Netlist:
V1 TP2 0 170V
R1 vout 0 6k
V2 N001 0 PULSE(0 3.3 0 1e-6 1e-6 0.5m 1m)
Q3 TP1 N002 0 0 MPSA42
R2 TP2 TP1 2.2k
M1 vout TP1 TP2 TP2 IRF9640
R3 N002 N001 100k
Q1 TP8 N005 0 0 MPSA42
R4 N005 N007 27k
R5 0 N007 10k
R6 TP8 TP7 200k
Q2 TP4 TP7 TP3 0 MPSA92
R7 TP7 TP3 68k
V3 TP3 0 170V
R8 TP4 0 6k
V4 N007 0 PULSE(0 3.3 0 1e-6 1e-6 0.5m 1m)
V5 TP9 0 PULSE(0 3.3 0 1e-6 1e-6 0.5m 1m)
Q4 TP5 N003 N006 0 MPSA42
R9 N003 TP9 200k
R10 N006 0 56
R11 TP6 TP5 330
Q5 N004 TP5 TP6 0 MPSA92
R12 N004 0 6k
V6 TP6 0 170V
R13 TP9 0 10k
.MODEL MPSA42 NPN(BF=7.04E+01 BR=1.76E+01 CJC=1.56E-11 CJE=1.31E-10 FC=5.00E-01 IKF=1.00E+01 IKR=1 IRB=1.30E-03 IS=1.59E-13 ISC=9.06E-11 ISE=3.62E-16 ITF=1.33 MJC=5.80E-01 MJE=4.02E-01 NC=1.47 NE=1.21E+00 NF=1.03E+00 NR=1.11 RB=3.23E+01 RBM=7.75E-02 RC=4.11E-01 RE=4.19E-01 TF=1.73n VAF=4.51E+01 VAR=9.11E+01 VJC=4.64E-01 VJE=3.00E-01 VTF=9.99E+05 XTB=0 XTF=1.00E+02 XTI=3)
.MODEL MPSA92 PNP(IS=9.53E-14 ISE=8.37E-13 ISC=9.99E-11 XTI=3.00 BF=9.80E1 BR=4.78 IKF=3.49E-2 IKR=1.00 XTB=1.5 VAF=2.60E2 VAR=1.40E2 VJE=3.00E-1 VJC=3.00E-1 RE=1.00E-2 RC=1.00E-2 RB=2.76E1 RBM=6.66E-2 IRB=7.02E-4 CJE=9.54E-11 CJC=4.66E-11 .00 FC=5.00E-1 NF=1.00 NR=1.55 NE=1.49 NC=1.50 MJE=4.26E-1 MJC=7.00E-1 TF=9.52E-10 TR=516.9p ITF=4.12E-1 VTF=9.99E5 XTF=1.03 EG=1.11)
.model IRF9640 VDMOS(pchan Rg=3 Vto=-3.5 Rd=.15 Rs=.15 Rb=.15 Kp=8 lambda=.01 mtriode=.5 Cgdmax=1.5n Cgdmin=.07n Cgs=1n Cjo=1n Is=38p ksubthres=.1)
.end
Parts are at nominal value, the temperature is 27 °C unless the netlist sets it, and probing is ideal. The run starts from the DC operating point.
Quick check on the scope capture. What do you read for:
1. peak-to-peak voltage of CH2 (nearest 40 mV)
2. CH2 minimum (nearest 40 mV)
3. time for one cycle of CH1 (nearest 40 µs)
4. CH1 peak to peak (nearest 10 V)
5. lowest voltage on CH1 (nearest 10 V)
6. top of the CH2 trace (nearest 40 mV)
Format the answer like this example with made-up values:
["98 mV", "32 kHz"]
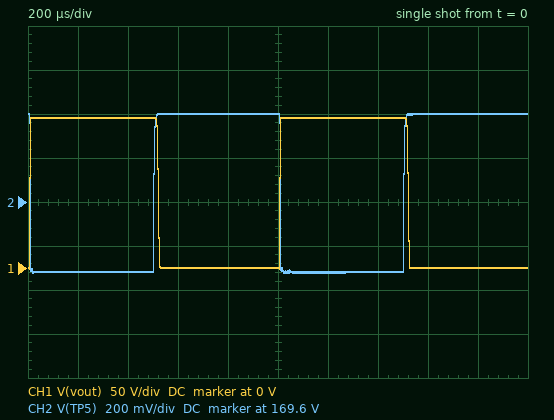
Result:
["720 mV", "169.28 V", "1.00 ms", "170 V", "0 V", "170.00 V"]
